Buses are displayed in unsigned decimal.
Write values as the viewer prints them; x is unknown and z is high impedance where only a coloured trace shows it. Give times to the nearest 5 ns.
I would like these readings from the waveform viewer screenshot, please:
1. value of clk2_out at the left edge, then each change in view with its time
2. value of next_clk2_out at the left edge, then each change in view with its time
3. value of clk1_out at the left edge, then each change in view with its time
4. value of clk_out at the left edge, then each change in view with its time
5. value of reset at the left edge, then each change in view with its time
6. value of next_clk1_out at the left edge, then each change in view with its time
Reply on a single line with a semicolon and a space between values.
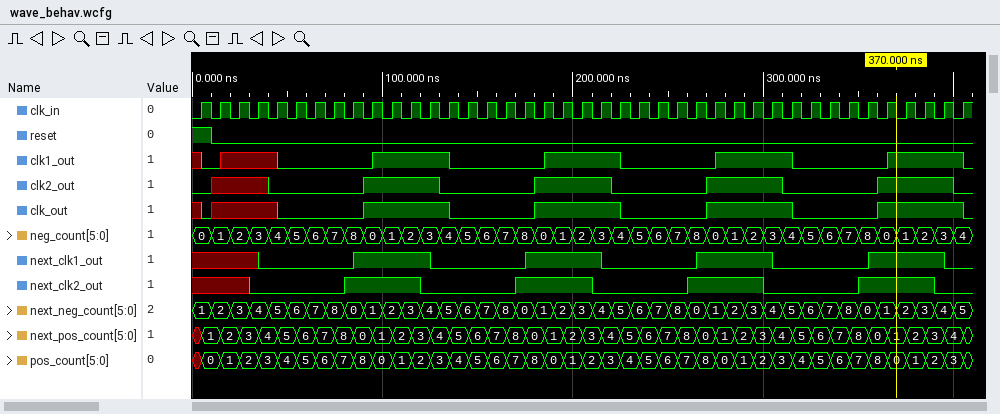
0, x at 10 ns, 0 at 40 ns, 1 at 90 ns, 0 at 130 ns, 1 at 180 ns, 0 at 220 ns, 1 at 270 ns, 0 at 310 ns, 1 at 360 ns, 0 at 400 ns; x, 0 at 30 ns, 1 at 80 ns, 0 at 120 ns, 1 at 170 ns, 0 at 210 ns, 1 at 260 ns, 0 at 300 ns, 1 at 350 ns, 0 at 390 ns; x, 0 at 5 ns, x at 15 ns, 0 at 45 ns, 1 at 95 ns, 0 at 135 ns, 1 at 185 ns, 0 at 225 ns, 1 at 275 ns, 0 at 315 ns, 1 at 365 ns, 0 at 405 ns; x, 0 at 5 ns, x at 10 ns, 0 at 45 ns, 1 at 90 ns, 0 at 135 ns, 1 at 180 ns, 0 at 225 ns, 1 at 270 ns, 0 at 315 ns, 1 at 360 ns, 0 at 405 ns; 1, 0 at 10 ns; x, 0 at 35 ns, 1 at 85 ns, 0 at 125 ns, 1 at 175 ns, 0 at 215 ns, 1 at 265 ns, 0 at 305 ns, 1 at 355 ns, 0 at 395 ns
